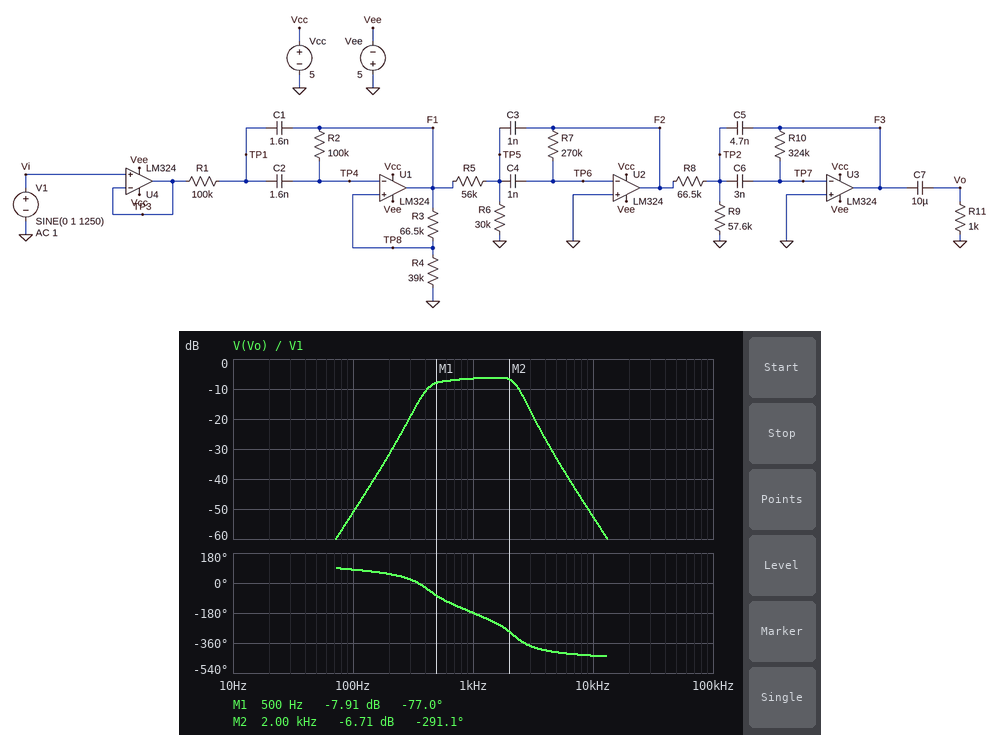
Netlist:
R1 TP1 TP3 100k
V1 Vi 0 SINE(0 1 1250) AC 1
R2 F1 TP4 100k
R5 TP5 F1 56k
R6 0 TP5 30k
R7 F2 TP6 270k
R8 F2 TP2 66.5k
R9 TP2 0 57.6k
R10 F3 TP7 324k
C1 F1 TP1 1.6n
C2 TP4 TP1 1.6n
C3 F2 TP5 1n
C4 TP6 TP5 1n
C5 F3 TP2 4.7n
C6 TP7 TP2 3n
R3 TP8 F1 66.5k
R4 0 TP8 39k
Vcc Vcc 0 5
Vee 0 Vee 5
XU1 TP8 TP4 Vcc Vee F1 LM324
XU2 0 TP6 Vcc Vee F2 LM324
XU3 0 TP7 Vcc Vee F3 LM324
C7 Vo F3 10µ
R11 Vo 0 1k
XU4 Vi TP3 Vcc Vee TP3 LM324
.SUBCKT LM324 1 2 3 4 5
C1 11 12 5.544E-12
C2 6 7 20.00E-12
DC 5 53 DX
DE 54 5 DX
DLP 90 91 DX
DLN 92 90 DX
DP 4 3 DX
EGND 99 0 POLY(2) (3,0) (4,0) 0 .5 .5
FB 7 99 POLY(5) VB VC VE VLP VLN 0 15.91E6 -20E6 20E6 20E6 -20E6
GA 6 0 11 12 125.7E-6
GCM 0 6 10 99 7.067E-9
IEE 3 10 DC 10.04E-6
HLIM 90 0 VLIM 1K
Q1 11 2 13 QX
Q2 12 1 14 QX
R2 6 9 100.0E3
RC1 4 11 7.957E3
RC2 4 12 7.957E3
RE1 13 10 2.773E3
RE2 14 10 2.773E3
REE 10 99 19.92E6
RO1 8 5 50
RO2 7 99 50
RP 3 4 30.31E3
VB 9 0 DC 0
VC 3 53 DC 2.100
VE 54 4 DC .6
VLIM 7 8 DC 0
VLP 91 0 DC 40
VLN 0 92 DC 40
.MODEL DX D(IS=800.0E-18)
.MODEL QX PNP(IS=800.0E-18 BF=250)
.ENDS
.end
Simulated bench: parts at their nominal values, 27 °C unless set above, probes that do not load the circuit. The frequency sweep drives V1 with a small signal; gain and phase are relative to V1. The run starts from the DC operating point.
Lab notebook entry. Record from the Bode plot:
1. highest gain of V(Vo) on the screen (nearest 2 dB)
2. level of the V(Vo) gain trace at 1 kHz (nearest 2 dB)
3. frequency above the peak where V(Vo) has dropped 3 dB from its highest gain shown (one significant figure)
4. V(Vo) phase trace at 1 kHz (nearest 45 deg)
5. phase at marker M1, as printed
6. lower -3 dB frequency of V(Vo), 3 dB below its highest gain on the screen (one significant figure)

-6 dB
-6 dB
2 kHz
-180 deg
-77.0 deg
400 Hz
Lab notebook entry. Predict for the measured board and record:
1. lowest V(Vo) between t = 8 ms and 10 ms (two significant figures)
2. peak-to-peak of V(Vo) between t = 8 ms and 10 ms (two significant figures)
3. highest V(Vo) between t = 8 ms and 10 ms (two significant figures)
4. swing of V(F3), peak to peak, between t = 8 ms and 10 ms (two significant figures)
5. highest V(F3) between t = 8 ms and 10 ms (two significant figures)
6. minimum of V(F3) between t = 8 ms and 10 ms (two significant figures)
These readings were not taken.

-480 mV
950 mV
480 mV
950 mV
470 mV
-480 mV
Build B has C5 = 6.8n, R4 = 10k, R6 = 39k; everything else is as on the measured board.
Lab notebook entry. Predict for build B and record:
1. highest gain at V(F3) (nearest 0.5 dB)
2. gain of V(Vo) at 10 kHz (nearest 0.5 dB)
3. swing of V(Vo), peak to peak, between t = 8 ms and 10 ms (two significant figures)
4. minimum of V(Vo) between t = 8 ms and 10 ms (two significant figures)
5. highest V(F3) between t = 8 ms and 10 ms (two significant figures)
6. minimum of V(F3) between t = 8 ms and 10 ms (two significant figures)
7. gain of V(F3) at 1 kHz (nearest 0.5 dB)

-12.5 dB
-58.5 dB
440 mV
-220 mV
210 mV
-230 mV
-13.5 dB
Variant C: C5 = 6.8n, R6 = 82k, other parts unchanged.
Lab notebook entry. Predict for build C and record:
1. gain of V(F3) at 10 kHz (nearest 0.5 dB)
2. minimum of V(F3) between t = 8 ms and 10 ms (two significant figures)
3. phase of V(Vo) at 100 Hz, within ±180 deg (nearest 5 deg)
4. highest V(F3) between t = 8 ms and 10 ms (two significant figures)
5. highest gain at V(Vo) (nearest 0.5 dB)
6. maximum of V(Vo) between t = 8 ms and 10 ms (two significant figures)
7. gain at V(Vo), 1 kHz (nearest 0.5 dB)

-56.0 dB
-590 mV
75 deg
580 mV
-4.5 dB
590 mV
-5.0 dB
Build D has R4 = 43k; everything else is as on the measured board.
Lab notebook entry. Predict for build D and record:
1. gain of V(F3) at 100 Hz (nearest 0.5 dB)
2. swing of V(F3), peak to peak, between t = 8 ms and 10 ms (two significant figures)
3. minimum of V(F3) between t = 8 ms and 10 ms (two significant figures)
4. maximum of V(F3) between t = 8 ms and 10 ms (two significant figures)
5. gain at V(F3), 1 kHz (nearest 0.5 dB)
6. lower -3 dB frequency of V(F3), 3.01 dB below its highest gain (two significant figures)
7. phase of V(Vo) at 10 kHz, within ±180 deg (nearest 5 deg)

-50.5 dB
1.0 V
-520 mV
510 mV
-6.0 dB
440 Hz
-75 deg
